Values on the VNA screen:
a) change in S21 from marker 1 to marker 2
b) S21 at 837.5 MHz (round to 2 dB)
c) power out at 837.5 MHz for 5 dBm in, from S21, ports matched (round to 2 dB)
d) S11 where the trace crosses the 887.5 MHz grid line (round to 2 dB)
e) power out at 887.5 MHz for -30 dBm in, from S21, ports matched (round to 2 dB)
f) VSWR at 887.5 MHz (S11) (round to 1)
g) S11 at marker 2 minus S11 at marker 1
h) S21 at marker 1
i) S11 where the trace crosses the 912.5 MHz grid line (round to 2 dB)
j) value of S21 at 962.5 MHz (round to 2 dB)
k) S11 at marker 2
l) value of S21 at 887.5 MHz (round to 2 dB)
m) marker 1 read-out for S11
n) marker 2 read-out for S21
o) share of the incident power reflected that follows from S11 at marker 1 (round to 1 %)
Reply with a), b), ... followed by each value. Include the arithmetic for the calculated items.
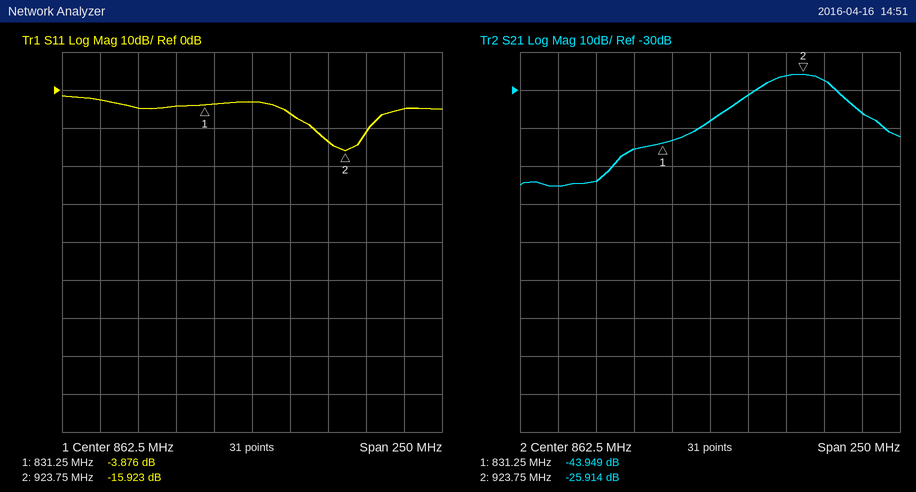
a) -25.914 − (-43.949) = 18.035 dB
b) -44 dB
c) 5 dBm + (-44 dB) = -38 dBm
d) -6 dB
e) -30 dBm + (-32 dB) = -62 dBm
f) |Γ| = 10^(-6/20) = 0.5012; VSWR = (1 + 0.5012)/(1 − 0.5012) ≈ 3
g) -15.923 − (-3.876) = -12.047 dB
h) -43.949 dB
i) -14 dB
j) -36 dB
k) -15.923 dB
l) -32 dB
m) -3.876 dB
n) -25.914 dB
o) 10^(-3.876/10) ≈ 41 %
